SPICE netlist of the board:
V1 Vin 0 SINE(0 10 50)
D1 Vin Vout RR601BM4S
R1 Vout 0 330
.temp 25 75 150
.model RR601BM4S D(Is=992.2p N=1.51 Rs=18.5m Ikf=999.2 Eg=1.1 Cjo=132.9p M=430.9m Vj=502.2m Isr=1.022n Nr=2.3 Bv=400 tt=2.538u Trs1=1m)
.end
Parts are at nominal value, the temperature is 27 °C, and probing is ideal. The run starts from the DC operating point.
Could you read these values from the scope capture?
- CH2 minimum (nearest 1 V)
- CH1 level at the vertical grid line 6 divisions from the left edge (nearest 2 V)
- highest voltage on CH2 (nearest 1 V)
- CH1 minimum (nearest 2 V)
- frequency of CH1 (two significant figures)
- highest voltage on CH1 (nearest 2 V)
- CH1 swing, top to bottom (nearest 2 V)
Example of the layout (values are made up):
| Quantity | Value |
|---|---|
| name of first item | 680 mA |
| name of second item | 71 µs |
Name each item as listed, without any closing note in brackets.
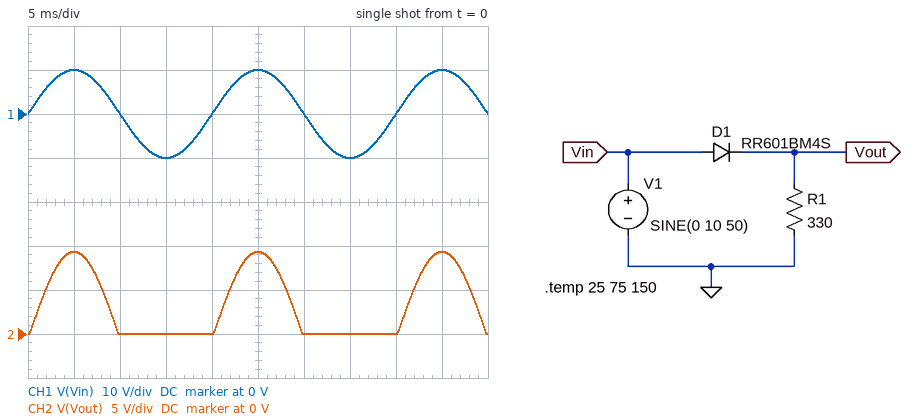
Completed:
| Quantity | Value |
|---|---|
| CH2 minimum | 0 V |
| CH1 level at the vertical grid line 6 divisions from the left edge | 0 V |
| highest voltage on CH2 | 9 V |
| CH1 minimum | -10 V |
| frequency of CH1 | 50 Hz |
| highest voltage on CH1 | 10 V |
| CH1 swing, top to bottom | 20 V |
